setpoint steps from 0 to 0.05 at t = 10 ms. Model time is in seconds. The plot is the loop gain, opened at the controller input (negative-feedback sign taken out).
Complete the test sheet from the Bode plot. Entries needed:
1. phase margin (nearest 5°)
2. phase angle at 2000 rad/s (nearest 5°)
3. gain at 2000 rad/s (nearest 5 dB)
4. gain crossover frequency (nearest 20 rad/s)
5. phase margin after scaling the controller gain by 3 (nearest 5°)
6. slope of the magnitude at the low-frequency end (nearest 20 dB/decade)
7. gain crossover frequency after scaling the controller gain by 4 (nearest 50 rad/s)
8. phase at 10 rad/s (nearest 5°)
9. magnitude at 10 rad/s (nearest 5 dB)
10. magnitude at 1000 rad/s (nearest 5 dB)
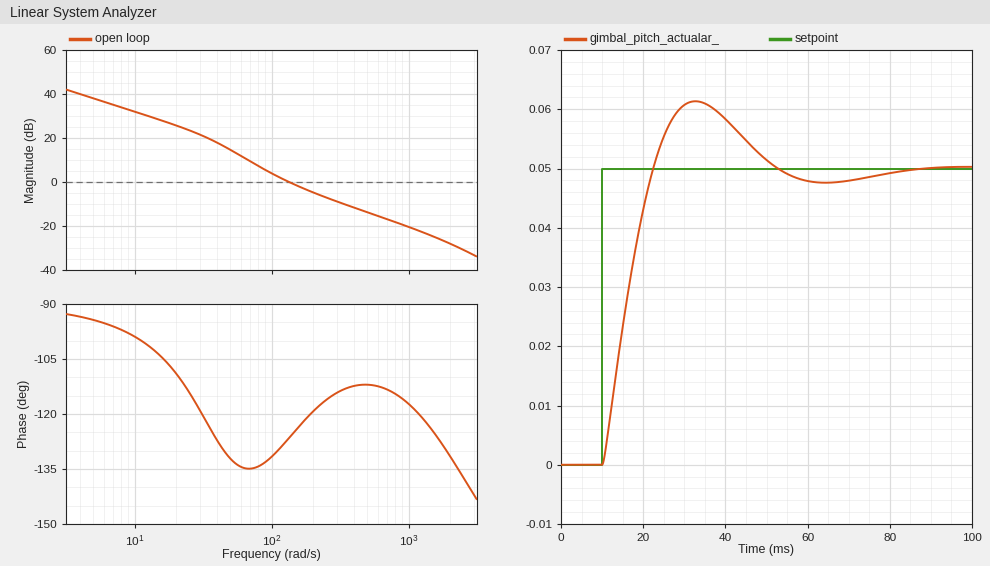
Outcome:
55°
-130°
-30 dB
140 rad/s
65°
-20 dB/decade
400 rad/s
-100°
30 dB
-20 dB
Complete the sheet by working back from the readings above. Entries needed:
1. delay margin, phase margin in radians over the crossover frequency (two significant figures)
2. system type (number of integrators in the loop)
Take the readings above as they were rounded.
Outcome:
0.0069 s
1
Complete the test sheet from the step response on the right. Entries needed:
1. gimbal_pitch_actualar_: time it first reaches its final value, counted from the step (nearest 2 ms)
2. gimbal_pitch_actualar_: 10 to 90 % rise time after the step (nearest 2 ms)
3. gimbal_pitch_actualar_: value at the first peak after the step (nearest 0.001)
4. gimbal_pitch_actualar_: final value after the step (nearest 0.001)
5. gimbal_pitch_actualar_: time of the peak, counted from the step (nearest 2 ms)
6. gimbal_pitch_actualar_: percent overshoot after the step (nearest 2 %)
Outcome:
12 ms
10 ms
0.061
0.050
22 ms
22 %
